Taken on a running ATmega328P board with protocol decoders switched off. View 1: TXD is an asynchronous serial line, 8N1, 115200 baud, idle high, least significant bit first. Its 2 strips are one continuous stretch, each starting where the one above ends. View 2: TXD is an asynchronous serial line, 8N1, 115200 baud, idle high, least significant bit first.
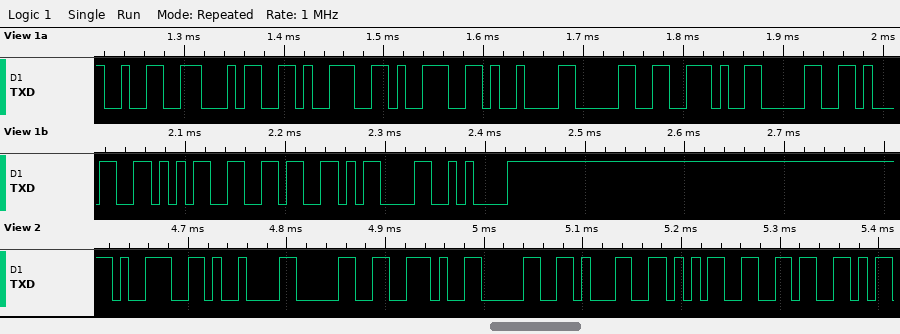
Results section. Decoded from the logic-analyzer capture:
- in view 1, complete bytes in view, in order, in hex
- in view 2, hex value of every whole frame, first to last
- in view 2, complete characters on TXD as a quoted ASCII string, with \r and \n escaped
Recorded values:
0x32 0x34 0x39 0x39 0x09 0x30 0x2E 0x30 0x31 0x35 0x36 0x0D 0x0A
39 09 30 2E 30 31 35 36
"9\t0.0156"
